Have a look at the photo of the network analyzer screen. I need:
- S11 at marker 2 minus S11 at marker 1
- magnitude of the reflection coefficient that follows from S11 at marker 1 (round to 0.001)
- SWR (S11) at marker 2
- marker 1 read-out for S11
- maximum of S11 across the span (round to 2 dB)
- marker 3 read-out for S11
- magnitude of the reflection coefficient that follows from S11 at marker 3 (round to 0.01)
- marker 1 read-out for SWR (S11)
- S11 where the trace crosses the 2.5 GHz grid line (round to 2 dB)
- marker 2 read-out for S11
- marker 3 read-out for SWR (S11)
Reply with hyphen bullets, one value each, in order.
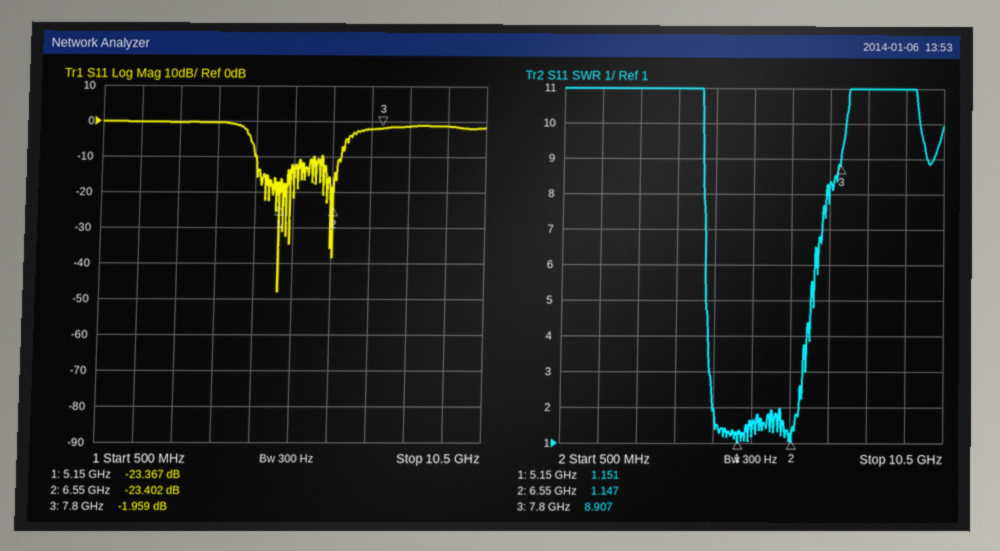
- -0.035 dB
- 0.068
- 1.147
- -23.367 dB
- 0 dB
- -1.959 dB
- 0.80
- 1.151
- 0 dB
- -23.402 dB
- 8.907
